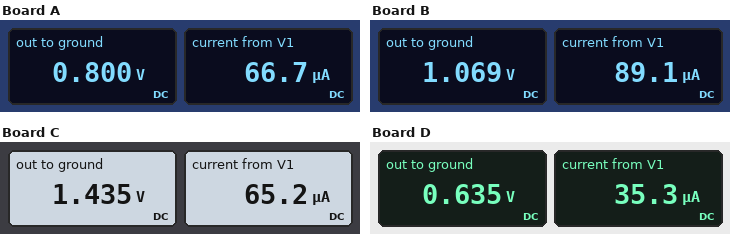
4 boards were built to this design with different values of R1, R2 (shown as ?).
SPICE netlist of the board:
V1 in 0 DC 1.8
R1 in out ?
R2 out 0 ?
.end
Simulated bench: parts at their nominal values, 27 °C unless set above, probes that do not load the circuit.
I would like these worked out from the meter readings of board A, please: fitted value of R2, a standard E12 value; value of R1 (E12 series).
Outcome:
12 kΩ
15 kΩ
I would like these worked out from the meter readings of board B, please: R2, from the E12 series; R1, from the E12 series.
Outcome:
12 kΩ
8.2 kΩ
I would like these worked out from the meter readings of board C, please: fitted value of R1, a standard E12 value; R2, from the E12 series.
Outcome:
5.6 kΩ
22 kΩ
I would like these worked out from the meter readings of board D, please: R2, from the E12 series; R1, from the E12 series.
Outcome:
18 kΩ
33 kΩ
